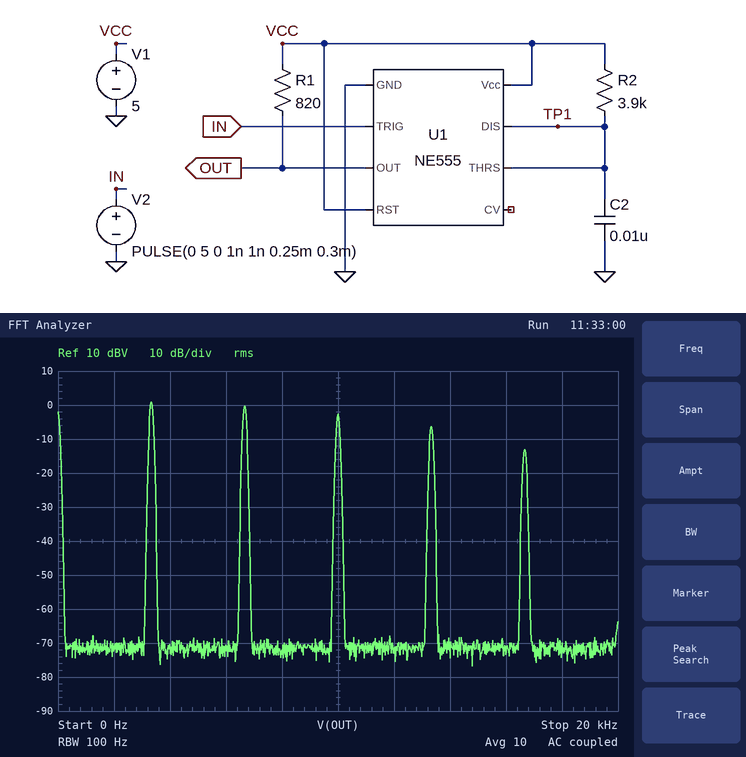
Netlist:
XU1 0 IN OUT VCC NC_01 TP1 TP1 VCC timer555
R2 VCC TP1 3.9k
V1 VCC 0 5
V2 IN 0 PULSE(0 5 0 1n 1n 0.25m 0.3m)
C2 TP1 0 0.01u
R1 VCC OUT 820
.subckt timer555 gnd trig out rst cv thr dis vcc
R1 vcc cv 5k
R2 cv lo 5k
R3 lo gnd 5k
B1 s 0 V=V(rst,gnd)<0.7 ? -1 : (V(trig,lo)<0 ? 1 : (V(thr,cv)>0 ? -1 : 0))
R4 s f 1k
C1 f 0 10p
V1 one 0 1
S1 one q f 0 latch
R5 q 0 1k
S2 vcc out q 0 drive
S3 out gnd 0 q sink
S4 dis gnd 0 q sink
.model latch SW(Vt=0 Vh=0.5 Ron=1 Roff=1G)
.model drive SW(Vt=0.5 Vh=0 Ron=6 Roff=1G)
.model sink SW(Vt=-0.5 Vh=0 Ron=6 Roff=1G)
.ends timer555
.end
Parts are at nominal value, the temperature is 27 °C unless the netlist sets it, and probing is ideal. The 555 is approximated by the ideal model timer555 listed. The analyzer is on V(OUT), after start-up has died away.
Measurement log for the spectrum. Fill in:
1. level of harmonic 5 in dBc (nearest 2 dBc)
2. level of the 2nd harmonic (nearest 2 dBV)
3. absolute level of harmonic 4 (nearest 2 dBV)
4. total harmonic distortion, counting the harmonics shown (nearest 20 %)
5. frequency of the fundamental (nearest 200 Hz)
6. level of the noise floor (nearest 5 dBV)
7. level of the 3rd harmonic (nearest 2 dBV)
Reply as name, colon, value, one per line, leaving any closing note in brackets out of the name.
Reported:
level of harmonic 5 in dBc: -14 dBc
level of the 2nd harmonic: 0 dBV
absolute level of harmonic 4: -6 dBV
total harmonic distortion, counting the harmonics shown: 120 %
frequency of the fundamental: 3.4 kHz
level of the noise floor: -70 dBV
level of the 3rd harmonic: -2 dBV
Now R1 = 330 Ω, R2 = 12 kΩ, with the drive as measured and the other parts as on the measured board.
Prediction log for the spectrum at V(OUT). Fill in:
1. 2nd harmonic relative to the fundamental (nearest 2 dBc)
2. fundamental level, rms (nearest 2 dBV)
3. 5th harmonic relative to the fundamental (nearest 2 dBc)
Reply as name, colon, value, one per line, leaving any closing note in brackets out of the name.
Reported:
2nd harmonic relative to the fundamental: -14 dBc
fundamental level, rms: 6 dBV
5th harmonic relative to the fundamental: -18 dBc
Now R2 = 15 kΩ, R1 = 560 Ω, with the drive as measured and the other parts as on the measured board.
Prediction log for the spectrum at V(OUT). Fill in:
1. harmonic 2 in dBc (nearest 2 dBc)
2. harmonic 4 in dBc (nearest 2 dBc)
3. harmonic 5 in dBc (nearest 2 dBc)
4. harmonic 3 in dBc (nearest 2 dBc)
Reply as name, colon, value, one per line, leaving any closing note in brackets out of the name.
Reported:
harmonic 2 in dBc: -16 dBc
harmonic 4 in dBc: -16 dBc
harmonic 5 in dBc: -16 dBc
harmonic 3 in dBc: -10 dBc
